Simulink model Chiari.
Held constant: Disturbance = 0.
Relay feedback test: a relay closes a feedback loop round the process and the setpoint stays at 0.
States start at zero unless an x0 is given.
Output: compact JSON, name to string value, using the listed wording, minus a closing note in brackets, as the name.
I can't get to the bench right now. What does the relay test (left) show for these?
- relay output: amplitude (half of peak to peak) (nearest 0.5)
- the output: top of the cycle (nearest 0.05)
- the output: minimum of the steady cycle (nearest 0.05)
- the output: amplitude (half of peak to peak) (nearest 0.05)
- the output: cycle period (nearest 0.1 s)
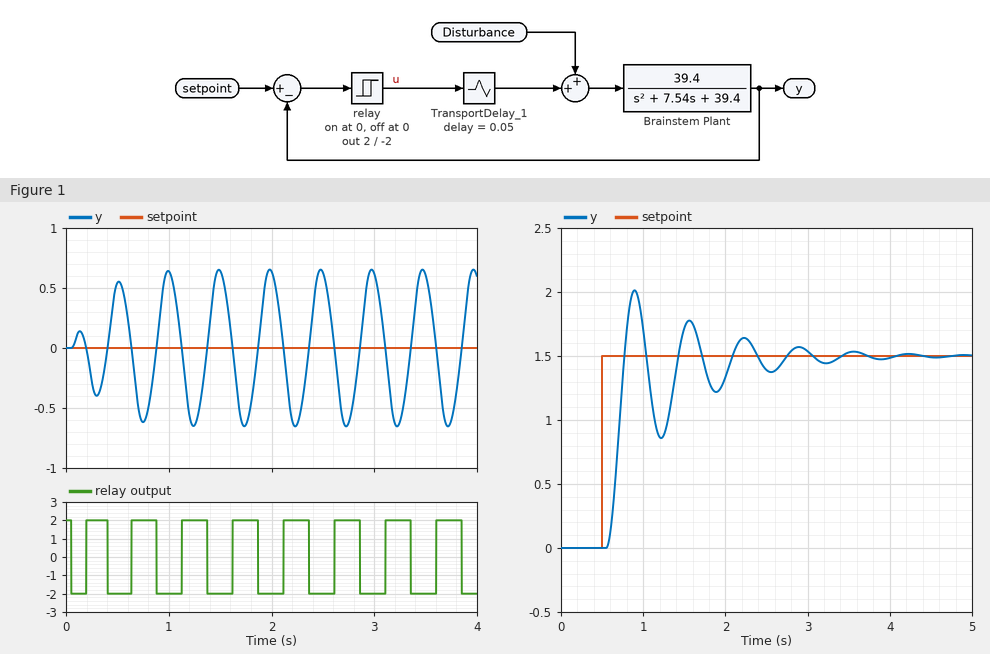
{"relay output: amplitude (half of peak to peak)": "2.0", "the output: top of the cycle": "0.65", "the output: minimum of the steady cycle": "-0.65", "the output: amplitude (half of peak to peak)": "0.65", "the output: cycle period": "0.5 s"}
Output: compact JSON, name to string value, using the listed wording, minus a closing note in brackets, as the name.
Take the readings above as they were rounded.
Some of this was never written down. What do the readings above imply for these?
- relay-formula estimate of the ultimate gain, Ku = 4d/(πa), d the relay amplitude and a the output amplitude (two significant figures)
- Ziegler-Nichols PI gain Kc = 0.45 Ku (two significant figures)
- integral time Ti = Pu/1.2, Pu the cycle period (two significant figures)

{"relay-formula estimate of the ultimate gain, Ku = 4d/(πa), d the relay amplitude and a the output amplitude": "3.9", "Ziegler-Nichols PI gain Kc = 0.45 Ku": "1.8", "integral time Ti = Pu/1.2, Pu the cycle period": "0.42 s"}
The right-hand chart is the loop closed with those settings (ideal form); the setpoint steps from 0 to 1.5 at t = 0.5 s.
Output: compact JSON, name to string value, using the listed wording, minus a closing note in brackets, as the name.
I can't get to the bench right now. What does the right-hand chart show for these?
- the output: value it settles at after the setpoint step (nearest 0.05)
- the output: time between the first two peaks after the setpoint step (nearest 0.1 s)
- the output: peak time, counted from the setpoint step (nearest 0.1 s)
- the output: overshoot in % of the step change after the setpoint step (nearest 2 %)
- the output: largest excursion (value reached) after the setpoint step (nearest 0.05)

{"the output: value it settles at after the setpoint step": "1.50", "the output: time between the first two peaks after the setpoint step": "0.7 s", "the output: peak time, counted from the setpoint step": "0.4 s", "the output: overshoot in % of the step change after the setpoint step": "34 %", "the output: largest excursion (value reached) after the setpoint step": "2.00"}
